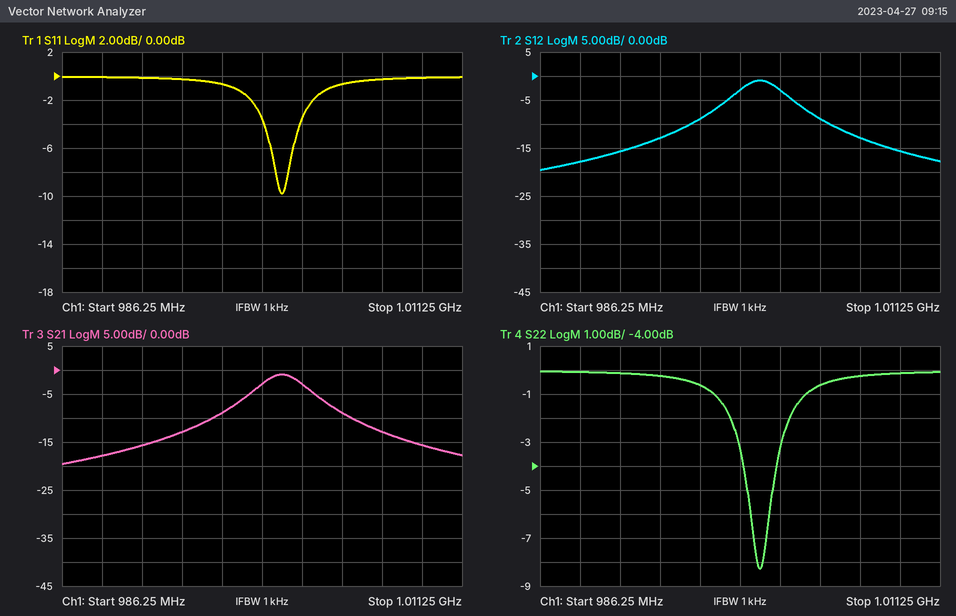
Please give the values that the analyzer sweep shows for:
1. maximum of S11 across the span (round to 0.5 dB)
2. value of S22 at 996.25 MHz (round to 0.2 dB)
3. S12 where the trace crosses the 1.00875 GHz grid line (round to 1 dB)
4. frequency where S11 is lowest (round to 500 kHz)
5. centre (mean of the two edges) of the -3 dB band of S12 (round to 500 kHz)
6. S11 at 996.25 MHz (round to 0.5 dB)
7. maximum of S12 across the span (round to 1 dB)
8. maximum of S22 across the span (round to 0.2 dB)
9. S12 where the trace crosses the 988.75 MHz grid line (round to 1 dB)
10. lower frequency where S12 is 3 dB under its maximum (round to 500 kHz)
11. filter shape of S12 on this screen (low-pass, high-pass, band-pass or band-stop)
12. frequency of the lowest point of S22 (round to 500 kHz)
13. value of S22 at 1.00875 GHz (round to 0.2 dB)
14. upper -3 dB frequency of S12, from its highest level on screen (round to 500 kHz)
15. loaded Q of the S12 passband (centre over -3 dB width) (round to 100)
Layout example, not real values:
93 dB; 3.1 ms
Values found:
0.0 dB; -0.6 dB; -16 dB; 1.0000 GHz; 1.0000 GHz; -0.5 dB; -1 dB; 0.0 dB; -18 dB; 998.5 MHz; band-pass; 1.0000 GHz; -0.2 dB; 1.0015 GHz; 300
